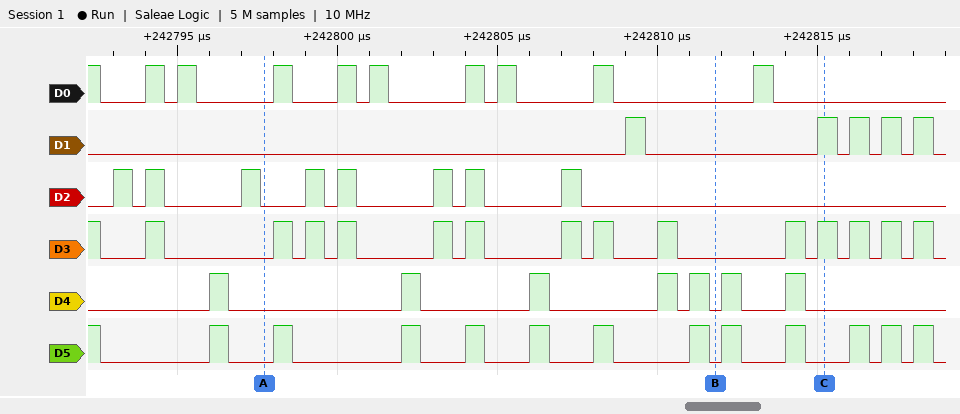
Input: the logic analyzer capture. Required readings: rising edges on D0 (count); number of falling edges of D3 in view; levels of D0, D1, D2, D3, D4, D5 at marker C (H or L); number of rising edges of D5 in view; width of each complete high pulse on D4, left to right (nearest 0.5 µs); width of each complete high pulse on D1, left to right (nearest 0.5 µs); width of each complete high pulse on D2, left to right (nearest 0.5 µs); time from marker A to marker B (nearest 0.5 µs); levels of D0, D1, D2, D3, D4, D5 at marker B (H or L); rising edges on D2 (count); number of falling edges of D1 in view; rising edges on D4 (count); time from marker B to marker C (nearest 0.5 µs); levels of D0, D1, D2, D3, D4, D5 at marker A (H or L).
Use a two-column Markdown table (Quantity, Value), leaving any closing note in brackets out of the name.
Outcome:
| Quantity | Value |
|---|---|
| rising edges on D0 | 9 |
| number of falling edges of D3 in view | 15 |
| levels of D0, D1, D2, D3, D4, D5 at marker C | D0=L, D1=H, D2=L, D3=H, D4=L, D5=L |
| number of rising edges of D5 in view | 12 |
| width of each complete high pulse on D4, left to right | 0.5 µs, 0.5 µs, 0.5 µs, 0.5 µs, 0.5 µs, 0.5 µs, 0.5 µs |
| width of each complete high pulse on D1, left to right | 0.5 µs, 0.5 µs, 0.5 µs, 0.5 µs, 0.5 µs |
| width of each complete high pulse on D2, left to right | 0.5 µs, 0.5 µs, 0.5 µs, 0.5 µs, 0.5 µs, 0.5 µs, 0.5 µs, 0.5 µs |
| time from marker A to marker B | 14 µs |
| levels of D0, D1, D2, D3, D4, D5 at marker B | D0=L, D1=L, D2=L, D3=L, D4=L, D5=L |
| rising edges on D2 | 8 |
| number of falling edges of D1 in view | 5 |
| rising edges on D4 | 7 |
| time from marker B to marker C | 3.5 µs |
| levels of D0, D1, D2, D3, D4, D5 at marker A | D0=L, D1=L, D2=L, D3=L, D4=L, D5=L |
